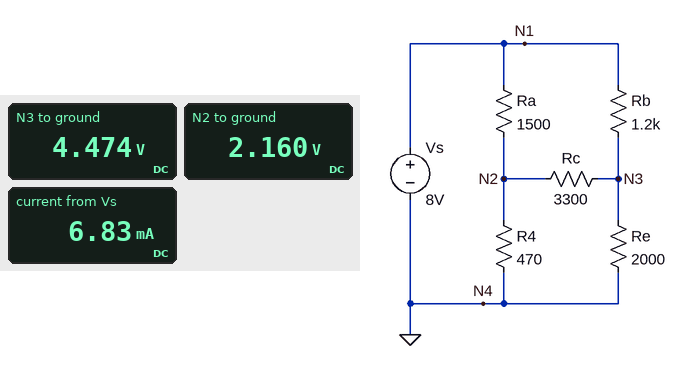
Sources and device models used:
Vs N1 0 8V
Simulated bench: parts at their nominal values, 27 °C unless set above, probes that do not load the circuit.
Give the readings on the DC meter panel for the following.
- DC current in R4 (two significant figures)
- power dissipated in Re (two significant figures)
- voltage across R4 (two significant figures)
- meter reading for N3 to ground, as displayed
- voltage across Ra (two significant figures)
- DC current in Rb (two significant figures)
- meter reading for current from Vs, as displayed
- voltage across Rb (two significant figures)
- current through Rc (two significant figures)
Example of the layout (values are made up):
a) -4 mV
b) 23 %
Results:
a) 4.6 mA
b) 10 mW
c) 2.2 V
d) 4.474 V
e) 5.8 V
f) 2.9 mA
g) 6.83 mA
h) 3.5 V
i) 700 µA
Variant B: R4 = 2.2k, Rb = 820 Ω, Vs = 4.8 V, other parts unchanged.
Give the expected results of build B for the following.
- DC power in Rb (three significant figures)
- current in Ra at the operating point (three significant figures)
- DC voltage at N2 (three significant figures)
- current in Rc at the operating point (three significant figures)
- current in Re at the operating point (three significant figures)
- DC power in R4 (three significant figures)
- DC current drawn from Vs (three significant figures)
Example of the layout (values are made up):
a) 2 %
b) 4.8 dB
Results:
a) 2.61 mW
b) 1.23 mA
c) 2.96 V
d) 115 µA
e) 1.67 mA
f) 3.97 mW
g) 3.01 mA
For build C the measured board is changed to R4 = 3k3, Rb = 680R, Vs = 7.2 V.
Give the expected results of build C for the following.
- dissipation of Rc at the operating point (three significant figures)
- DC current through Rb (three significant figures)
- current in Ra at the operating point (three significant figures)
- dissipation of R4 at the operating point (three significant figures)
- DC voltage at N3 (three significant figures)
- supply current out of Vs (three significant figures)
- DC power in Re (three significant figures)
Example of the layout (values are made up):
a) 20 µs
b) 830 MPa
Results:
a) 25.2 µW
b) 2.75 mA
c) 1.44 mA
d) 7.70 mW
e) 5.33 V
f) 4.19 mA
g) 14.2 mW
